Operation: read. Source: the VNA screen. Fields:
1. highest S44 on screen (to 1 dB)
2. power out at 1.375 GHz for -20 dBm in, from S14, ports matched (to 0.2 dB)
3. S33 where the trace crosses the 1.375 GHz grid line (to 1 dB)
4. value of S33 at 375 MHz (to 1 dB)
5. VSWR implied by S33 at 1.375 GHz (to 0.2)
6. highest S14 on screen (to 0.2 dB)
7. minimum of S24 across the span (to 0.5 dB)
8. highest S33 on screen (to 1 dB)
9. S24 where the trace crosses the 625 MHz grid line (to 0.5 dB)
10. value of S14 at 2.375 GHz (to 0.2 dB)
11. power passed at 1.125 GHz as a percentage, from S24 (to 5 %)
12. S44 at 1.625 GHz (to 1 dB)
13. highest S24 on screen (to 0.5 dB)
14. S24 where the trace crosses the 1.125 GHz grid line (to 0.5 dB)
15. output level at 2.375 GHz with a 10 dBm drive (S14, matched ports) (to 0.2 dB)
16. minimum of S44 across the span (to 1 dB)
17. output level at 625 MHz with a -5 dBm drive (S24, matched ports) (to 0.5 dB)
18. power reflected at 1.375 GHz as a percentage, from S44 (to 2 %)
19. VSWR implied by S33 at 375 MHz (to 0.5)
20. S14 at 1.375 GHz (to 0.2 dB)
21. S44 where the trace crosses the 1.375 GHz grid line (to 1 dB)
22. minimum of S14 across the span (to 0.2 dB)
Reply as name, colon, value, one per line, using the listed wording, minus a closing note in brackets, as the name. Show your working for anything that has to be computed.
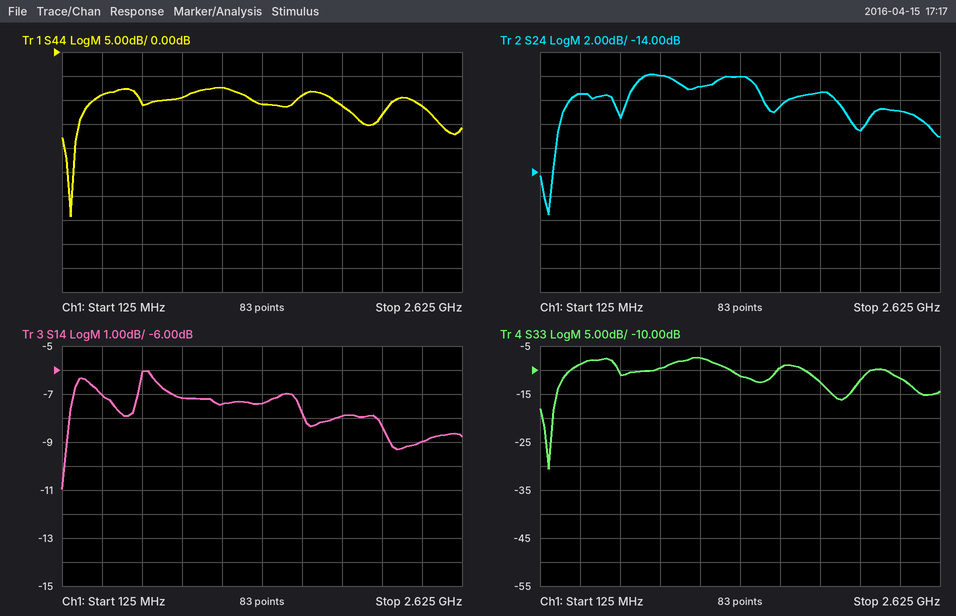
highest S44 on screen: -7 dB
power out at 1.375 GHz for -20 dBm in, from S14, ports matched: -20 dBm + (-7.4 dB) = -27.4 dBm
S33 where the trace crosses the 1.375 GHz grid line: -11 dB
value of S33 at 375 MHz: -9 dB
VSWR implied by S33 at 1.375 GHz: |Γ| = 10^(-11/20) = 0.2818; VSWR = (1 + 0.2818)/(1 − 0.2818) ≈ 1.8
highest S14 on screen: -6.0 dB
minimum of S24 across the span: -17.5 dB
highest S33 on screen: -7 dB
S24 where the trace crosses the 625 MHz grid line: -9.5 dB
value of S14 at 2.375 GHz: -9.0 dB
power passed at 1.125 GHz as a percentage, from S24: 10^(-7/10) ≈ 20 %
S44 at 1.625 GHz: -9 dB
highest S24 on screen: -6.0 dB
S24 where the trace crosses the 1.125 GHz grid line: -7.0 dB
output level at 2.375 GHz with a 10 dBm drive (S14, matched ports): 10 dBm + (-9.0 dB) = 1.0 dBm
minimum of S44 across the span: -34 dB
output level at 625 MHz with a -5 dBm drive (S24, matched ports): -5 dBm + (-9.5 dB) = -14.5 dBm
power reflected at 1.375 GHz as a percentage, from S44: 10^(-11/10) ≈ 8 %
VSWR implied by S33 at 375 MHz: |Γ| = 10^(-9/20) = 0.3548; VSWR = (1 + 0.3548)/(1 − 0.3548) ≈ 2.10, so 2.0 to the nearest 0.5
S14 at 1.375 GHz: -7.4 dB
S44 where the trace crosses the 1.375 GHz grid line: -11 dB
minimum of S14 across the span: -11.0 dB
